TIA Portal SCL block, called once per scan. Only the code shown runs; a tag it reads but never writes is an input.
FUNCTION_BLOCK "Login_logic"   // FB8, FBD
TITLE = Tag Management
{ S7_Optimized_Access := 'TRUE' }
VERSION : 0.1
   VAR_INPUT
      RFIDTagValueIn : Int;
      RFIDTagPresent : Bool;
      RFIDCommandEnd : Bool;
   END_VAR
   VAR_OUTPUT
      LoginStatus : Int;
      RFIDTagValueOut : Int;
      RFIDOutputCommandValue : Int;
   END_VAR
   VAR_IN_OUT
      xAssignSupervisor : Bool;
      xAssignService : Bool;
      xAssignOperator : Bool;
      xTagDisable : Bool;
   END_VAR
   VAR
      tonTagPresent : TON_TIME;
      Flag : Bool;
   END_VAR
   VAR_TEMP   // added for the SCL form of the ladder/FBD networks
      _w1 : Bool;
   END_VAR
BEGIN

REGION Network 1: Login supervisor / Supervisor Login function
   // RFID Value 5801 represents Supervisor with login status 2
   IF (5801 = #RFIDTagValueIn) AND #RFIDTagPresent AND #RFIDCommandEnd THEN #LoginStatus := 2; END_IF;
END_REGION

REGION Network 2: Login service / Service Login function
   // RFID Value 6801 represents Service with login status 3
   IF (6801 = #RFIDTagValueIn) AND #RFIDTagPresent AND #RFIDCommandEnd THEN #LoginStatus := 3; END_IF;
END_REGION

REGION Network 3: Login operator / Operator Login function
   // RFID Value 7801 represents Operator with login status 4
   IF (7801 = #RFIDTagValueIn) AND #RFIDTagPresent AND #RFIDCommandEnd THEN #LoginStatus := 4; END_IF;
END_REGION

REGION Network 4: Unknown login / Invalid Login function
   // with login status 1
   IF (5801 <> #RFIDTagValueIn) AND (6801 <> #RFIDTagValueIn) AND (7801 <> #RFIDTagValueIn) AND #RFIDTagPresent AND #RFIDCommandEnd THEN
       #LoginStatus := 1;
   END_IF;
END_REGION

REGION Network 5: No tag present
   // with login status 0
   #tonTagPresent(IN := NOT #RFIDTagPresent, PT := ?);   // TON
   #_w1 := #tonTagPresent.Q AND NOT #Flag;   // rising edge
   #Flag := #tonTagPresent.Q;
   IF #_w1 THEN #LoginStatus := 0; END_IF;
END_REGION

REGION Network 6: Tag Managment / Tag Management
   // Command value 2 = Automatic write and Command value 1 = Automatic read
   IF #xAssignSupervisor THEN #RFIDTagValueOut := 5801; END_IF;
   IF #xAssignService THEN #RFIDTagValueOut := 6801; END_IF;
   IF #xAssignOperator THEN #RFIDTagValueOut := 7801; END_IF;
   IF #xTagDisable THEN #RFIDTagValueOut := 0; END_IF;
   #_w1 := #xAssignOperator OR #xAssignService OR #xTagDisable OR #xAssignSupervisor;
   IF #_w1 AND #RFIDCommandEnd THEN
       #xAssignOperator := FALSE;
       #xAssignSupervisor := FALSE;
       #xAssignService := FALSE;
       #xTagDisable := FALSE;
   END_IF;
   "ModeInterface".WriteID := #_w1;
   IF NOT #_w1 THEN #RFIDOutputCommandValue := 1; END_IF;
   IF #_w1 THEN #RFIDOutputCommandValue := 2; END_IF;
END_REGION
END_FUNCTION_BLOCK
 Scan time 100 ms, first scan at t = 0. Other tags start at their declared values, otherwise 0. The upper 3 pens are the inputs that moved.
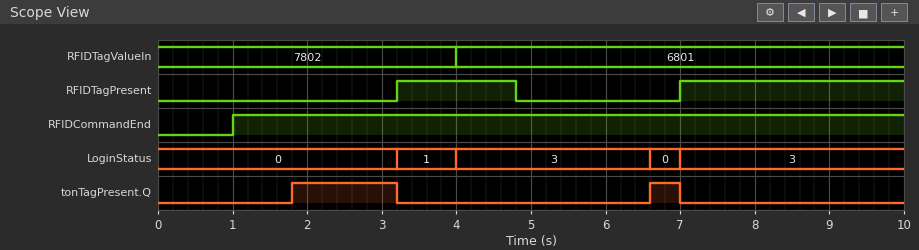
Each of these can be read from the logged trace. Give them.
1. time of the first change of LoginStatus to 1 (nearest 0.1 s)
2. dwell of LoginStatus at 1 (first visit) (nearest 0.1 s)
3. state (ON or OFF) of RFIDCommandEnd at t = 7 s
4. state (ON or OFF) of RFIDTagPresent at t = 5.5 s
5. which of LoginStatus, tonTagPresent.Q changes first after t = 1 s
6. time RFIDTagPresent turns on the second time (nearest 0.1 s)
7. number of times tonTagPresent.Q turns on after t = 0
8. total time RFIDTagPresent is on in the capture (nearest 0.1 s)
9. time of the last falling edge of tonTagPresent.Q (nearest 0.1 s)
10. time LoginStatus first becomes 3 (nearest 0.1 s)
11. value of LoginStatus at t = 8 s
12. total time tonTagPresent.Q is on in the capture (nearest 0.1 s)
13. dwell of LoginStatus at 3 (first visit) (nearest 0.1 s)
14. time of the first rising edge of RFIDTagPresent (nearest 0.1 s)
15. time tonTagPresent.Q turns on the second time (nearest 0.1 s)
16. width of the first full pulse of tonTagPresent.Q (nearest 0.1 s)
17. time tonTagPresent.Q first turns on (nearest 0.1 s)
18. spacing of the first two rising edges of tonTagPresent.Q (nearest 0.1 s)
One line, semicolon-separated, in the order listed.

3.2 s; 0.8 s; ON; OFF; tonTagPresent.Q; 7.0 s; 2; 4.6 s; 7.0 s; 4.0 s; 3; 1.8 s; 2.6 s; 3.2 s; 6.6 s; 1.4 s; 1.8 s; 4.8 s
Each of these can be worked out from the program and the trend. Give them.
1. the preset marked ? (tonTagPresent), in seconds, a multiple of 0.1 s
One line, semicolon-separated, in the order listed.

1.8 s
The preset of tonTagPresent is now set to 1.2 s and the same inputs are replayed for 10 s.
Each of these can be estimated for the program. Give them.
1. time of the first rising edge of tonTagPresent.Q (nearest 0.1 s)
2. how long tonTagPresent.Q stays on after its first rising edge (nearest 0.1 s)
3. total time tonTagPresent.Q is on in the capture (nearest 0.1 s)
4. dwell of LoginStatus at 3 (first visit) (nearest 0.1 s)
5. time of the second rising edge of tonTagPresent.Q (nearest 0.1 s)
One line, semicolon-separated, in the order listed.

1.2 s; 2.0 s; 3.0 s; 2.0 s; 6.0 s
